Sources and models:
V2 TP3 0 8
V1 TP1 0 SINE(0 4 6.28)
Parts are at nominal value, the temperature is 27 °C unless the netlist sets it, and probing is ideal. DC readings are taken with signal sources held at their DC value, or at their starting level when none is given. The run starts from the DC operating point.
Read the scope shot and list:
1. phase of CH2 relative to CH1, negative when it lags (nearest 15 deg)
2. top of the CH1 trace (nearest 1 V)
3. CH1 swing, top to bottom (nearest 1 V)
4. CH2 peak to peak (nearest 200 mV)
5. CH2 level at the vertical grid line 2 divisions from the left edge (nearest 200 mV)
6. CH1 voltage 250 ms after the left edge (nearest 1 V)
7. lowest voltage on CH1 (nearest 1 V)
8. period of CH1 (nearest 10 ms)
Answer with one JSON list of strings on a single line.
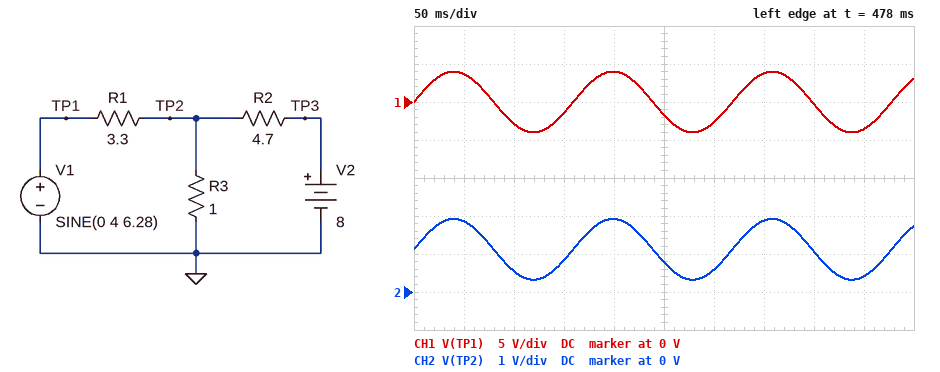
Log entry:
["0 deg", "4 V", "8 V", "1.6 V", "600 mV", "-2 V", "-4 V", "160 ms"]
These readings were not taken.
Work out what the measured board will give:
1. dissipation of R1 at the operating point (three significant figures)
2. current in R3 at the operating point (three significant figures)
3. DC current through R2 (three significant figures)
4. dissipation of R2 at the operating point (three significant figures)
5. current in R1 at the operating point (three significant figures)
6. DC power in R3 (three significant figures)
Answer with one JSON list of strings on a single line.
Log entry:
["382 mW", "1.12 A", "1.46 A", "10.1 W", "340 mA", "1.26 W"]
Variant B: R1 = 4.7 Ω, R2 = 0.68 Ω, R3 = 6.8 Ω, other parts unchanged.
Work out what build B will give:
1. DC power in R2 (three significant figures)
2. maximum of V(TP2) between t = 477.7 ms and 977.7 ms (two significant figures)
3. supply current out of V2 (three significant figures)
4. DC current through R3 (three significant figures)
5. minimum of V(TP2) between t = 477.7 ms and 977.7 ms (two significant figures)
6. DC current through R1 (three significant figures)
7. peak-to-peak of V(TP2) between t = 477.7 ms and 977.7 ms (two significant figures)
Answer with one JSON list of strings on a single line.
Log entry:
["3.64 W", "6.9 V", "2.31 A", "945 mA", "6.0 V", "1.37 A", "930 mV"]
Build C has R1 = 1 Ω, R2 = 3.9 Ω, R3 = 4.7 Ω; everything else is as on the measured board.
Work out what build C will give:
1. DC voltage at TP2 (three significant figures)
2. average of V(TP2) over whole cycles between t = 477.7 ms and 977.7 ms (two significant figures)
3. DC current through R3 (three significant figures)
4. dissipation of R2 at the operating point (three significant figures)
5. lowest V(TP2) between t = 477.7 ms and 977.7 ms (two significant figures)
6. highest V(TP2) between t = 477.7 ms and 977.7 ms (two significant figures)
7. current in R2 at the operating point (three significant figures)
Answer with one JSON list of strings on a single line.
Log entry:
["1.40 V", "1.4 V", "297 mA", "11.2 W", "-1.3 V", "4.1 V", "1.69 A"]
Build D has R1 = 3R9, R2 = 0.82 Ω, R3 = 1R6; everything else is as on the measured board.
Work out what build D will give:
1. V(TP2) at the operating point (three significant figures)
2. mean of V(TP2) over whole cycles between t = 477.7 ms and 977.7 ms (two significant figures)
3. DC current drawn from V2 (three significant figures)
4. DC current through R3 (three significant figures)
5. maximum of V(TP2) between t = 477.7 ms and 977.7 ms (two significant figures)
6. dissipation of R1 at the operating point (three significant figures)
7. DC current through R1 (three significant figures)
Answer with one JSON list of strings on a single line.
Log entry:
["4.64 V", "4.6 V", "4.09 A", "2.90 A", "5.1 V", "5.53 W", "1.19 A"]
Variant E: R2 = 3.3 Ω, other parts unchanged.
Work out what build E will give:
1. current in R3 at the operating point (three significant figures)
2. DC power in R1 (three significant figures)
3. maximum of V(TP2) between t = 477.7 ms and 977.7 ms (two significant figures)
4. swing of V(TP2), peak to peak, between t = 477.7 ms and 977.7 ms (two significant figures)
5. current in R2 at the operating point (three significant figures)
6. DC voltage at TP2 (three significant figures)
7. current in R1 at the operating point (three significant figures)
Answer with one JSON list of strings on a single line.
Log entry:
["1.51 A", "690 mW", "2.3 V", "1.5 V", "1.97 A", "1.51 V", "457 mA"]
